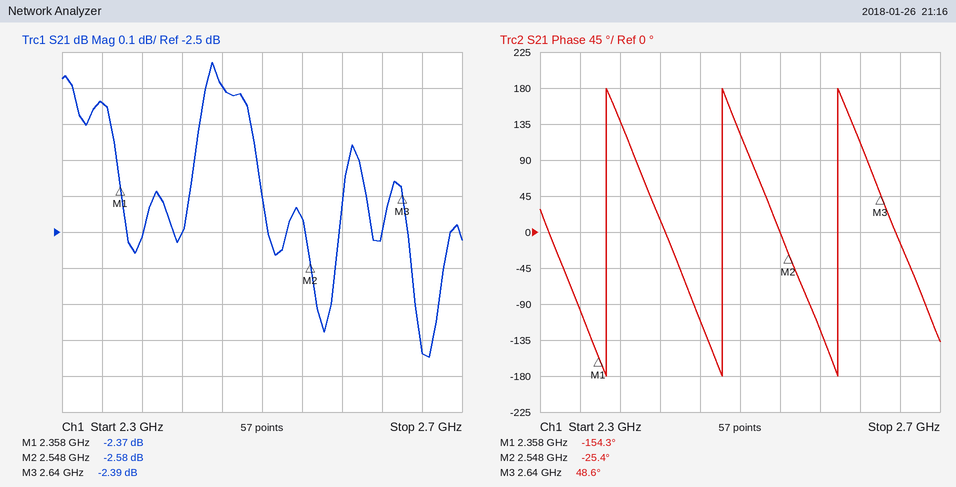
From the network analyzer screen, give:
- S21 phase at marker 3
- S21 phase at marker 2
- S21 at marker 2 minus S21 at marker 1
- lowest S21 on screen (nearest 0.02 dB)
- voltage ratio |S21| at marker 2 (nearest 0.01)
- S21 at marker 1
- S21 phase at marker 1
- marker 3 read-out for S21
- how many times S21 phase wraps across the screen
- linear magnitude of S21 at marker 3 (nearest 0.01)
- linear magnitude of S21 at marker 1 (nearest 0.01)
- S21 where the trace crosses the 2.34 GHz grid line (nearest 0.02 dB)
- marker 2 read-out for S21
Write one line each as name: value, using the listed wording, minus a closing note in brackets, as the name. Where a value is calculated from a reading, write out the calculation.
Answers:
S21 phase at marker 3: 48.6°
S21 phase at marker 2: -25.4°
S21 at marker 2 minus S21 at marker 1: -2.58 − (-2.37) = -0.21 dB
lowest S21 on screen: -2.84 dB
voltage ratio |S21| at marker 2: 10^(-2.58/20) ≈ 0.74
S21 at marker 1: -2.37 dB
S21 phase at marker 1: -154.3°
marker 3 read-out for S21: -2.39 dB
how many times S21 phase wraps across the screen: 3
linear magnitude of S21 at marker 3: 10^(-2.39/20) ≈ 0.76
linear magnitude of S21 at marker 1: 10^(-2.37/20) ≈ 0.76
S21 where the trace crosses the 2.34 GHz grid line: -2.14 dB
marker 2 read-out for S21: -2.58 dB
